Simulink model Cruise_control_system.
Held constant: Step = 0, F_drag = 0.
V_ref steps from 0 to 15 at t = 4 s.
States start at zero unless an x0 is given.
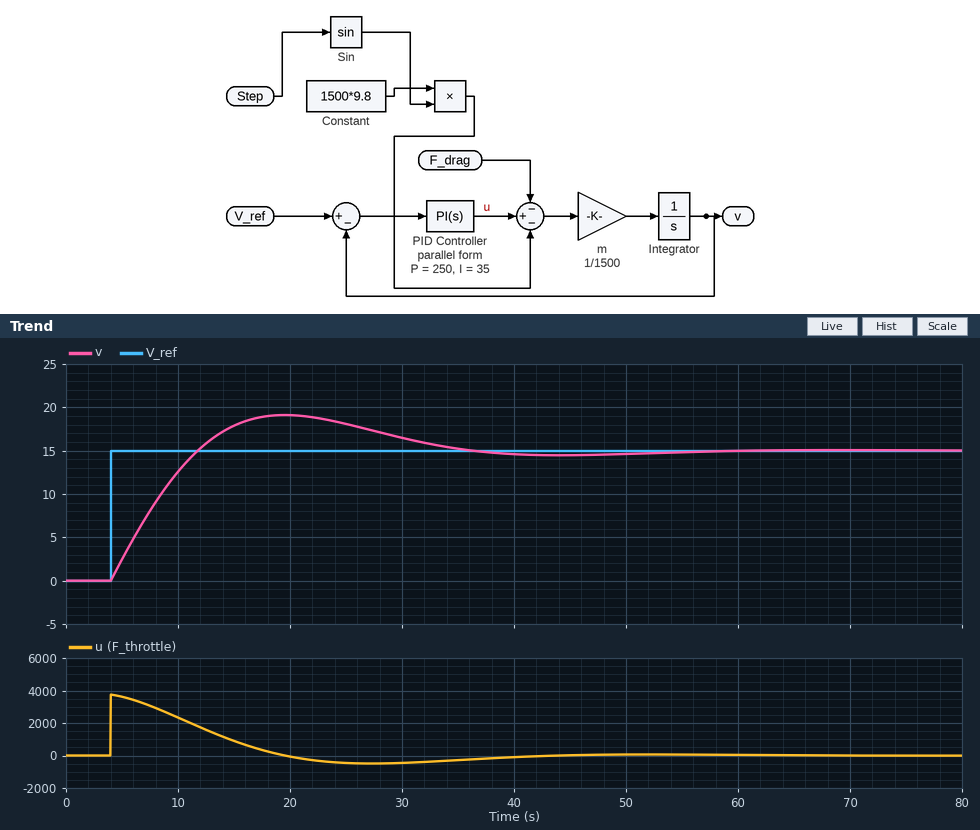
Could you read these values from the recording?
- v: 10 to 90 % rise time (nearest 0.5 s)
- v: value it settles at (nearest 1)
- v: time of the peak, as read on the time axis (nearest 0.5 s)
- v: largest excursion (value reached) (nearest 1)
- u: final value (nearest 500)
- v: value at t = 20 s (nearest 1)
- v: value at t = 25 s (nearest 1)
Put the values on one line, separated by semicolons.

6.0 s; 15; 19.5 s; 19; 0; 19; 18
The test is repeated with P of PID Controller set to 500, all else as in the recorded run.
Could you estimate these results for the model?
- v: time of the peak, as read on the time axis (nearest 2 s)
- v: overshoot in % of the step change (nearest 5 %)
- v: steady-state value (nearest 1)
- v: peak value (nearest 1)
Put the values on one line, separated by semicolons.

16 s; 10 %; 15; 17
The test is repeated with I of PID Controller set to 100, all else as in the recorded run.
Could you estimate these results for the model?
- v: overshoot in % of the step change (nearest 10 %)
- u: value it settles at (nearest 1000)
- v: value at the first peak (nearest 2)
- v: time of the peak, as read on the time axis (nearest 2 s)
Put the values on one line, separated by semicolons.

40 %; 0; 22; 14 s
